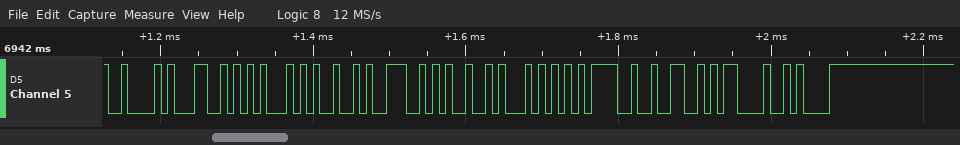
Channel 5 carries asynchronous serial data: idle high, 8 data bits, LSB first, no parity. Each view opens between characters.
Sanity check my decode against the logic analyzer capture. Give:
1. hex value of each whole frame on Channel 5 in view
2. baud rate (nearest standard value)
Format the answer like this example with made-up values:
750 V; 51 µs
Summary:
42, 4C, 45, 49, 4E, 49, 54, 3D, 32, 0D, 0A; 115200 baud
